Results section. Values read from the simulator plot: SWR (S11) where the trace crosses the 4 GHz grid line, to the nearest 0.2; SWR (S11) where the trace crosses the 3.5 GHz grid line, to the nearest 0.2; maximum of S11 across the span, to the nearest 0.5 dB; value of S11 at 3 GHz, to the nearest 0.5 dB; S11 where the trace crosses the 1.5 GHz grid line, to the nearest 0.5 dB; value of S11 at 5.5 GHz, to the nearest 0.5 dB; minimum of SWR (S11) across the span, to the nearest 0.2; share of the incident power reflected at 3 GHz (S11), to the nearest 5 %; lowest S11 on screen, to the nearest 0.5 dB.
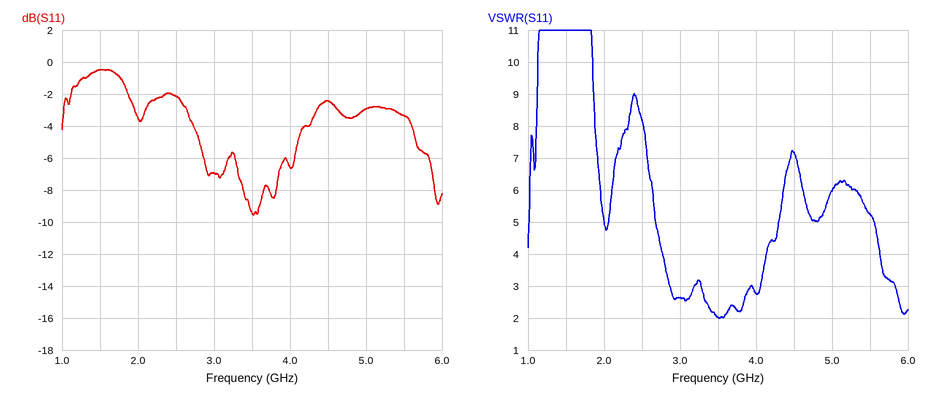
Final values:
2.8
2.0
-0.5 dB
-7.0 dB
-0.5 dB
-3.5 dB
2.0
20 %
-9.5 dB
